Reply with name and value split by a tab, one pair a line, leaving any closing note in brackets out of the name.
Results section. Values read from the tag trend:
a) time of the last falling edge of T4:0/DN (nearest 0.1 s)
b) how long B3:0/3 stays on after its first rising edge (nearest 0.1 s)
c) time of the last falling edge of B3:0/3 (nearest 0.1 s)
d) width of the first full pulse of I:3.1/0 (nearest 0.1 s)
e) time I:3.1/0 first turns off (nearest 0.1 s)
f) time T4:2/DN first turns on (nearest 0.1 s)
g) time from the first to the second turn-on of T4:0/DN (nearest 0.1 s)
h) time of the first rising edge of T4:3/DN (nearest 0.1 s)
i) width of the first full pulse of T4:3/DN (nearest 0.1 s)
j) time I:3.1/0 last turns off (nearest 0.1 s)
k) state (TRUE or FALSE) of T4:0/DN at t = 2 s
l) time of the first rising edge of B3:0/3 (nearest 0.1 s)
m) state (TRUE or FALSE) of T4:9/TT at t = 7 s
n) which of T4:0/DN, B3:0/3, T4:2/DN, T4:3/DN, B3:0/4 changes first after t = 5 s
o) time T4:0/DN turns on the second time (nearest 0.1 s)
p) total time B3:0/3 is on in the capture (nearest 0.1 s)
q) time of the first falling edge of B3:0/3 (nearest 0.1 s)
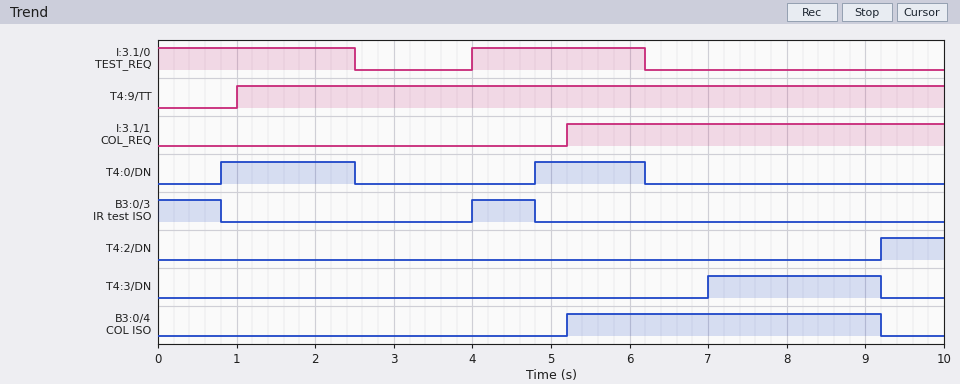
time of the last falling edge of T4:0/DN	6.2 s
how long B3:0/3 stays on after its first rising edge	0.8 s
time of the last falling edge of B3:0/3	4.8 s
width of the first full pulse of I:3.1/0	2.2 s
time I:3.1/0 first turns off	2.5 s
time T4:2/DN first turns on	9.2 s
time from the first to the second turn-on of T4:0/DN	4.0 s
time of the first rising edge of T4:3/DN	7.0 s
width of the first full pulse of T4:3/DN	2.2 s
time I:3.1/0 last turns off	6.2 s
state (TRUE or FALSE) of T4:0/DN at t = 2 s	TRUE
time of the first rising edge of B3:0/3	4.0 s
state (TRUE or FALSE) of T4:9/TT at t = 7 s	TRUE
which of T4:0/DN, B3:0/3, T4:2/DN, T4:3/DN, B3:0/4 changes first after t = 5 s	B3:0/4
time T4:0/DN turns on the second time	4.8 s
total time B3:0/3 is on in the capture	1.6 s
time of the first falling edge of B3:0/3	0.8 s
